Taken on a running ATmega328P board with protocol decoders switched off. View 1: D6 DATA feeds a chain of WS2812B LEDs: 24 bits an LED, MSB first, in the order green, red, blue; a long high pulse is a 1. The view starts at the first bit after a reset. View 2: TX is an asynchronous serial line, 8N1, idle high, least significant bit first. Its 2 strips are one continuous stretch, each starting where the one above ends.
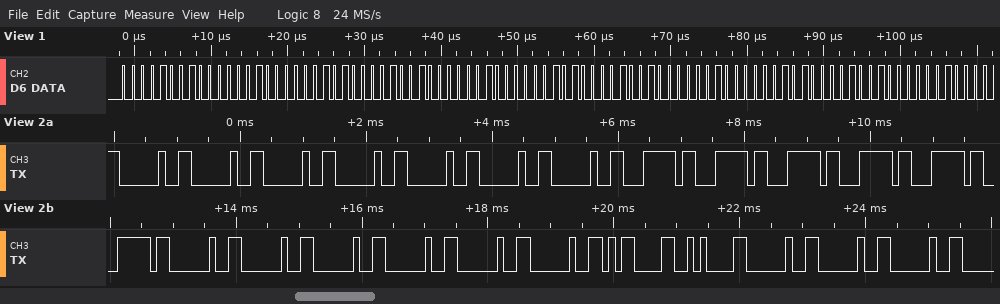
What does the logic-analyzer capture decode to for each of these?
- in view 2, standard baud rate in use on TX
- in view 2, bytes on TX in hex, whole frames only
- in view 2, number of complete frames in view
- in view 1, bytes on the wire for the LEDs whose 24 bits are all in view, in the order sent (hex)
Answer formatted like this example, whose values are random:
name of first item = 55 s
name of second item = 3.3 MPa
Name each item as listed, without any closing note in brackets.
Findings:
in view 2, standard baud rate in use on TX = 9600 baud
in view 2, bytes on TX in hex, whole frames only = 20 20 20 20 20 20 20 7C 7C 7C 7C 7C 7C 20 20 20 20 20 20 0D 0A 20 20 20
in view 2, number of complete frames in view = 24
in view 1, bytes on the wire for the LEDs whose 24 bits are all in view, in the order sent = 09 02 05 09 02 05 09 02 05
